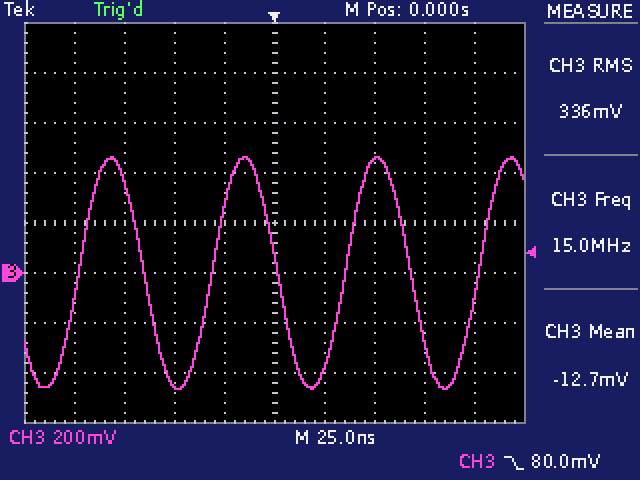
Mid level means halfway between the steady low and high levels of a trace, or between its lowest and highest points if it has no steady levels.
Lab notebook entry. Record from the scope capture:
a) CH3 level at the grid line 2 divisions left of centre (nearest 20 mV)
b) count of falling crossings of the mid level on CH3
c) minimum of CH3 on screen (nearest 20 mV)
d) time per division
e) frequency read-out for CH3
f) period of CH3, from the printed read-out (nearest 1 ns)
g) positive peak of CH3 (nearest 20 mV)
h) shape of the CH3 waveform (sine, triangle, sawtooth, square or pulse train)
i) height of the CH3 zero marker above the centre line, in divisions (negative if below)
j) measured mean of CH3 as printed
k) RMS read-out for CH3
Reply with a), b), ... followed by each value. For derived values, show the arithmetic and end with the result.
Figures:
a) -440 mV
b) 3
c) -460 mV
d) 25 ns
e) 15.0 MHz
f) 1 / 15.0 MHz ≈ 67 ns
g) 460 mV
h) sine
i) -1.0 div
j) -12.7 mV
k) 336 mV
